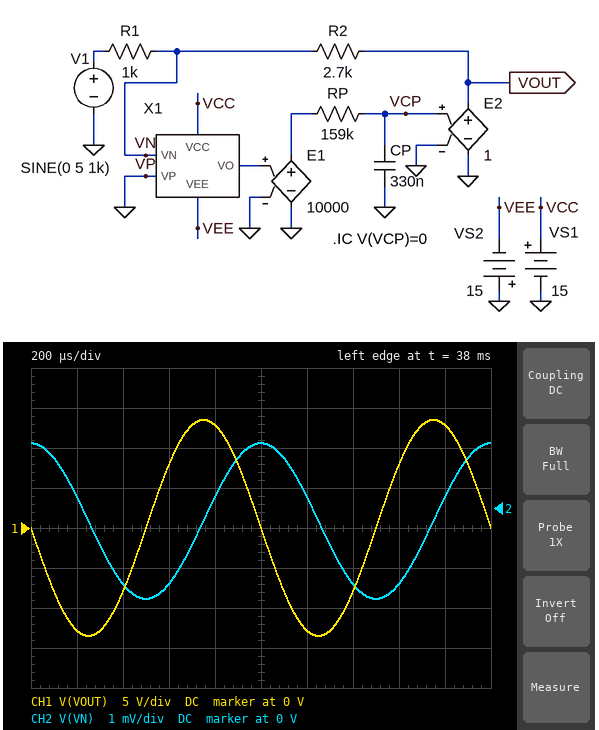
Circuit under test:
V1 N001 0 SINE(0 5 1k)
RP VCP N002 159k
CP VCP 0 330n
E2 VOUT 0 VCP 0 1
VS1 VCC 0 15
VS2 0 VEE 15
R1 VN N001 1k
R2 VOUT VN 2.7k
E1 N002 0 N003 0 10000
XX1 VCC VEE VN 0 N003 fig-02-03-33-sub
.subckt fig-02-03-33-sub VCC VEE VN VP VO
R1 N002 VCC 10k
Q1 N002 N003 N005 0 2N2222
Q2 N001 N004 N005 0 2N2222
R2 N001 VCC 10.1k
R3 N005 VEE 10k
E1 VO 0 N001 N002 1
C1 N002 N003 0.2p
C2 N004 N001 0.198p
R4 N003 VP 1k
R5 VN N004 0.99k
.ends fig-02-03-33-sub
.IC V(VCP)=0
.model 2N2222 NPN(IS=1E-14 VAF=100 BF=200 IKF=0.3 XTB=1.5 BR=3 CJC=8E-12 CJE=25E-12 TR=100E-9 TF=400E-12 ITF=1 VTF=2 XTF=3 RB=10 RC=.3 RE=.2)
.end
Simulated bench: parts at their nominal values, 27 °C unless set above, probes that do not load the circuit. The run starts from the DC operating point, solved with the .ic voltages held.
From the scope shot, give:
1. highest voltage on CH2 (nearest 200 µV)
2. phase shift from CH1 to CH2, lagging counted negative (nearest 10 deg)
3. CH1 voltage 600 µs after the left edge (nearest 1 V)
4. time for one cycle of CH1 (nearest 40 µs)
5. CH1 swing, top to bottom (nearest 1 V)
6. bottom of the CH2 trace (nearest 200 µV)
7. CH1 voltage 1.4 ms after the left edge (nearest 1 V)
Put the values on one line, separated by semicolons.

1.6 mV; -90 deg; 8 V; 1.00 ms; 27 V; -2.2 mV; -8 V
